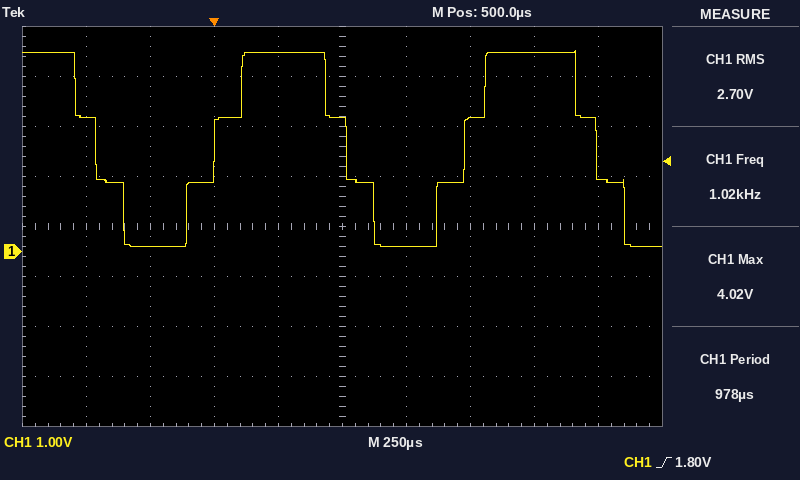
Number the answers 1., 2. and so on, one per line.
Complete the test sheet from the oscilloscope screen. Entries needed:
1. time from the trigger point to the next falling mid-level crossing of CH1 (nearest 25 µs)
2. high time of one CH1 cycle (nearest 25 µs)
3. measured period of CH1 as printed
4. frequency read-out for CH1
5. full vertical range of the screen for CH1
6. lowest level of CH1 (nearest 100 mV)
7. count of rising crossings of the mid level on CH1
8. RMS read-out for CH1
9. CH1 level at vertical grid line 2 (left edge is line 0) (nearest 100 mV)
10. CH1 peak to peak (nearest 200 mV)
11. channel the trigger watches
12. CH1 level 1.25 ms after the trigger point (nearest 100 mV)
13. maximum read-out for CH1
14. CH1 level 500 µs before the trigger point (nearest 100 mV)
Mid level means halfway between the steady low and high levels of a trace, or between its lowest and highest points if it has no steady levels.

1. 525 µs
2. 525 µs
3. 978 µs
4. 1.02 kHz
5. 8 V
6. 100 mV
7. 2
8. 2.70 V
9. 100 mV
10. 4.0 V
11. CH1
12. 4.0 V
13. 4.02 V
14. 2.7 V
